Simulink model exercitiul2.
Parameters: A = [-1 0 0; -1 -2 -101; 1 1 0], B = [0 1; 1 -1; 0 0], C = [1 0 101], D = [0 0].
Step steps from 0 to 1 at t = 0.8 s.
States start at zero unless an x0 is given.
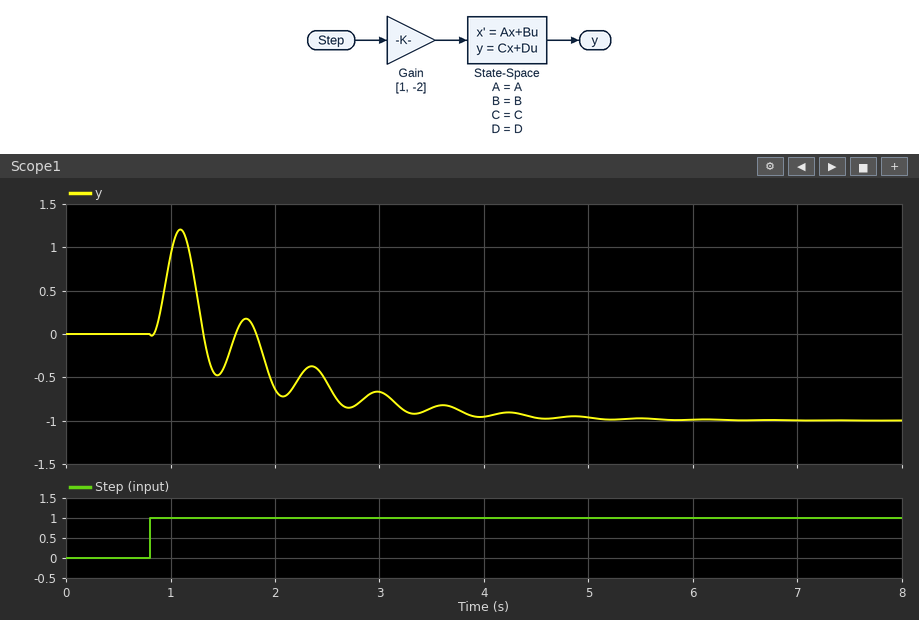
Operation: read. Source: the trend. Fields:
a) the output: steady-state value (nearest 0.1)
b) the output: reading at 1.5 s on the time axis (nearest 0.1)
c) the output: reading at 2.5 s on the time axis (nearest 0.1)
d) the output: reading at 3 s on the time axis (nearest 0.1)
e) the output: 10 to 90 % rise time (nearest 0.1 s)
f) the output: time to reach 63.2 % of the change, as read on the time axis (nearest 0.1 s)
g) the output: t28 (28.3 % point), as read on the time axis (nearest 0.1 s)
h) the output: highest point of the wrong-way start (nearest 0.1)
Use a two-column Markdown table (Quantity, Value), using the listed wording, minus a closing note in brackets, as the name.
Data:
| Quantity | Value |
|---|---|
| the output: steady-state value | -1.0 |
| the output: reading at 1.5 s on the time axis | -0.4 |
| the output: reading at 2.5 s on the time axis | -0.6 |
| the output: reading at 3 s on the time axis | -0.7 |
| the output: 10 to 90 % rise time | 1.9 s |
| the output: time to reach 63.2 % of the change, as read on the time axis | 2.0 s |
| the output: t28 (28.3 % point), as read on the time axis | 1.4 s |
| the output: highest point of the wrong-way start | 1.2 |
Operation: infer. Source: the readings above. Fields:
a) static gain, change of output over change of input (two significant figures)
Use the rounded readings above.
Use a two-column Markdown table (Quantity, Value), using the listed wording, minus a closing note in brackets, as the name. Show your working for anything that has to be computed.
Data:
| Quantity | Value |
|---|---|
| static gain, change of output over change of input | (-1 - 0) / (1 - 0) = -1.0 |
